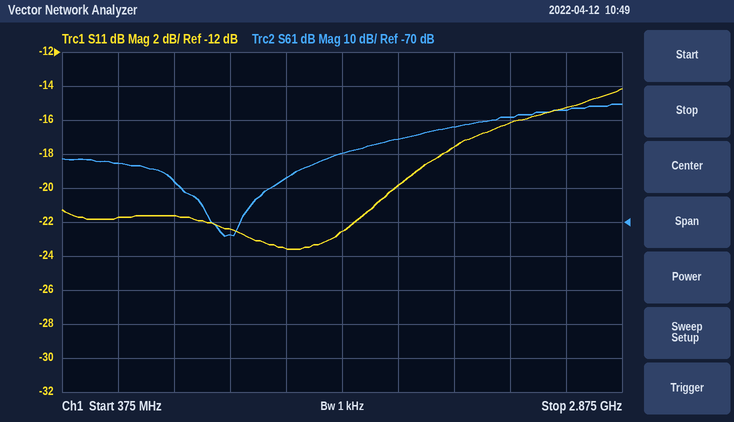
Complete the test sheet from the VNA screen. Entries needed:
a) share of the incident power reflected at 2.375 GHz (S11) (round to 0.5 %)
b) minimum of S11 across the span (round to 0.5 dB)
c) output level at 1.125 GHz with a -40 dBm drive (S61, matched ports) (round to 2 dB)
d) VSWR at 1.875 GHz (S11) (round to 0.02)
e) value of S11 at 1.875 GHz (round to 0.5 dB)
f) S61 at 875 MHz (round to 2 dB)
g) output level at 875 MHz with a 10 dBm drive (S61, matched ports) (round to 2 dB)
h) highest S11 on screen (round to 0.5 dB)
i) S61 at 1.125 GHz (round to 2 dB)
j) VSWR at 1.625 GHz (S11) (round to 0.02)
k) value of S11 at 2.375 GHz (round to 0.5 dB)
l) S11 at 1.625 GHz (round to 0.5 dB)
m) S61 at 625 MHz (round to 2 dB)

2.5 %
-23.5 dB
-114 dBm
1.22
-20.0 dB
-58 dB
-48 dBm
-14.0 dB
-74 dB
1.16
-16.0 dB
-22.5 dB
-52 dB
